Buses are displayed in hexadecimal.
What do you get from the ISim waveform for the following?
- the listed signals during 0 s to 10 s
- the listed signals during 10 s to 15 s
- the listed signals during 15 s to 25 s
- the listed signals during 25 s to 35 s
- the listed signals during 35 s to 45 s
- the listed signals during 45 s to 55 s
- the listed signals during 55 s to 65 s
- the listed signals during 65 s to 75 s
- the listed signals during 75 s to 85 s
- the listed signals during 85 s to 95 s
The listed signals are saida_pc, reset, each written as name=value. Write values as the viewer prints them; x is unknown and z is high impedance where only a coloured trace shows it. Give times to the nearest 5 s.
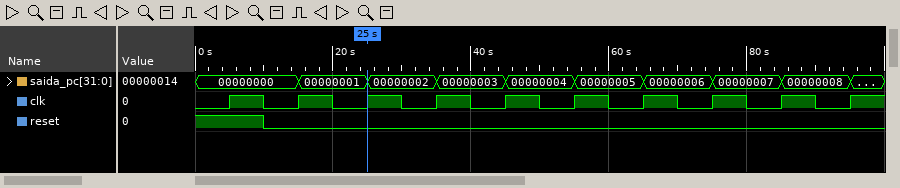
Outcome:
saida_pc=00000000, reset=1
saida_pc=00000000, reset=0
saida_pc=00000001, reset=0
saida_pc=00000002, reset=0
saida_pc=00000003, reset=0
saida_pc=00000004, reset=0
saida_pc=00000005, reset=0
saida_pc=00000006, reset=0
saida_pc=00000007, reset=0
saida_pc=00000008, reset=0
